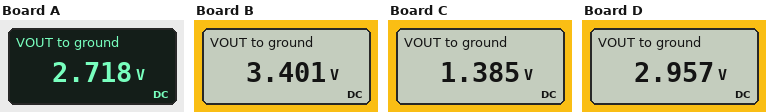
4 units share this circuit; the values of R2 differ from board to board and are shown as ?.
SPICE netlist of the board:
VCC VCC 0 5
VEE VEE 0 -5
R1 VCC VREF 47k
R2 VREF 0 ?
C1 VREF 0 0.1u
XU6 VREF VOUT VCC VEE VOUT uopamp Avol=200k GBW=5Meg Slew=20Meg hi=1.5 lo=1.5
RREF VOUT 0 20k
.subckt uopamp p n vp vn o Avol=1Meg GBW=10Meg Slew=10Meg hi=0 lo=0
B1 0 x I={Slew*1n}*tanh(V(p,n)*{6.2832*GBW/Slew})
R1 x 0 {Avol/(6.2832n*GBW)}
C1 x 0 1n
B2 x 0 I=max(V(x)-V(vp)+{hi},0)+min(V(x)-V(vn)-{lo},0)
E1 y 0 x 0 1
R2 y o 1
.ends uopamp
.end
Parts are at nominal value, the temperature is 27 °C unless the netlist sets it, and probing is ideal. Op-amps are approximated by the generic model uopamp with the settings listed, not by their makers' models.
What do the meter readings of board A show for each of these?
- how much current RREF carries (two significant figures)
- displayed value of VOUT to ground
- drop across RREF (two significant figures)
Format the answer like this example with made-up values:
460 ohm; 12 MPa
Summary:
140 µA; 2.718 V; 2.7 V
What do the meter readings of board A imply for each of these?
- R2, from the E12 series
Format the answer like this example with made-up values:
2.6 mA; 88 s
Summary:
56 kΩ
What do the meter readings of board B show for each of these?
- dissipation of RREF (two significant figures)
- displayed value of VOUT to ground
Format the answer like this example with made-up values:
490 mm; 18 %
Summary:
580 µW; 3.401 V
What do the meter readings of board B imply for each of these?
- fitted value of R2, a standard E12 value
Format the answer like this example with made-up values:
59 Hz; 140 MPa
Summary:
100 kΩ
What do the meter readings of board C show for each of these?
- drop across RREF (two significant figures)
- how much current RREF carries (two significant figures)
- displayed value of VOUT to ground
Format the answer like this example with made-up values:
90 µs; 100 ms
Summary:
1.4 V; 69 µA; 1.385 V
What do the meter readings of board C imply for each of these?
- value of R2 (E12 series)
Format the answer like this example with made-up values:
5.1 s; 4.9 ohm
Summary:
18 kΩ
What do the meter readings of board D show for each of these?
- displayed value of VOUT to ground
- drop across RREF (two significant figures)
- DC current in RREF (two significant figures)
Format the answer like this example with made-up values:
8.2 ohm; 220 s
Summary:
2.957 V; 3.0 V; 150 µA
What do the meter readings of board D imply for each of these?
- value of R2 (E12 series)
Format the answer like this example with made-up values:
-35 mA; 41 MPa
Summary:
68 kΩ
